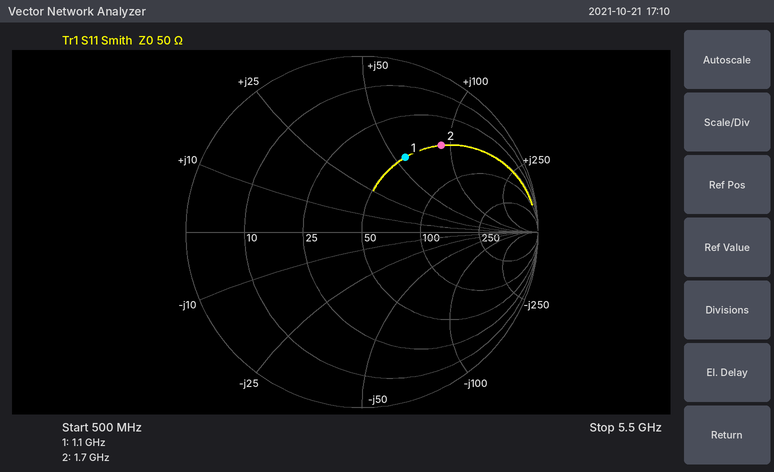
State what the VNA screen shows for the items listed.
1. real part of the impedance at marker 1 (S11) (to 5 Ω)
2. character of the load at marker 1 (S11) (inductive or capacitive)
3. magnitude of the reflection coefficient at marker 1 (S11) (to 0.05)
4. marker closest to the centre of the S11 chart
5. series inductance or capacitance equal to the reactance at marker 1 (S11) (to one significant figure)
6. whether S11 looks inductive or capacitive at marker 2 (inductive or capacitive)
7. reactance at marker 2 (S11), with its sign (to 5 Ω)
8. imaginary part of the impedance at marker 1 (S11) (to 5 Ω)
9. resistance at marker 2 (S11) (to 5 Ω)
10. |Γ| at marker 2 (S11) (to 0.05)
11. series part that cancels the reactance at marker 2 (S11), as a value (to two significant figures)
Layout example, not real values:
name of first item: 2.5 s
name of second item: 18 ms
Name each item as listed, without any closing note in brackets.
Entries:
real part of the impedance at marker 1 (S11): 50 Ω
character of the load at marker 1 (S11): inductive
magnitude of the reflection coefficient at marker 1 (S11): 0.50
marker closest to the centre of the S11 chart: marker 1
series inductance or capacitance equal to the reactance at marker 1 (S11): 8 nH
whether S11 looks inductive or capacitive at marker 2: inductive
reactance at marker 2 (S11), with its sign: +90 Ω
imaginary part of the impedance at marker 1 (S11): +55 Ω
resistance at marker 2 (S11): 50 Ω
|Γ| at marker 2 (S11): 0.65
series part that cancels the reactance at marker 2 (S11), as a value: 1.0 pF
